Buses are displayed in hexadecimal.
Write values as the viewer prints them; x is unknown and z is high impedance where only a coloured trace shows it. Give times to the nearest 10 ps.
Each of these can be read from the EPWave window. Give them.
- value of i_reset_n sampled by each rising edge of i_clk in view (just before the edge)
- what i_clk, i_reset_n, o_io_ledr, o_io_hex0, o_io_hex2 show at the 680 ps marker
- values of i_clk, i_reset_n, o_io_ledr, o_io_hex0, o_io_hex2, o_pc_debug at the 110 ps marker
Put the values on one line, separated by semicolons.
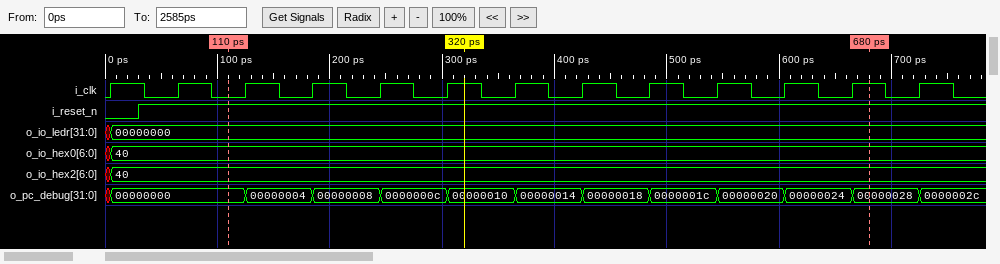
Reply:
0 1 1 1 1 1 1 1 1 1 1 1 1; i_clk=1, i_reset_n=1, o_io_ledr=00000000, o_io_hex0=40, o_io_hex2=40; i_clk=0, i_reset_n=1, o_io_ledr=00000000, o_io_hex0=40, o_io_hex2=40, o_pc_debug=00000000
